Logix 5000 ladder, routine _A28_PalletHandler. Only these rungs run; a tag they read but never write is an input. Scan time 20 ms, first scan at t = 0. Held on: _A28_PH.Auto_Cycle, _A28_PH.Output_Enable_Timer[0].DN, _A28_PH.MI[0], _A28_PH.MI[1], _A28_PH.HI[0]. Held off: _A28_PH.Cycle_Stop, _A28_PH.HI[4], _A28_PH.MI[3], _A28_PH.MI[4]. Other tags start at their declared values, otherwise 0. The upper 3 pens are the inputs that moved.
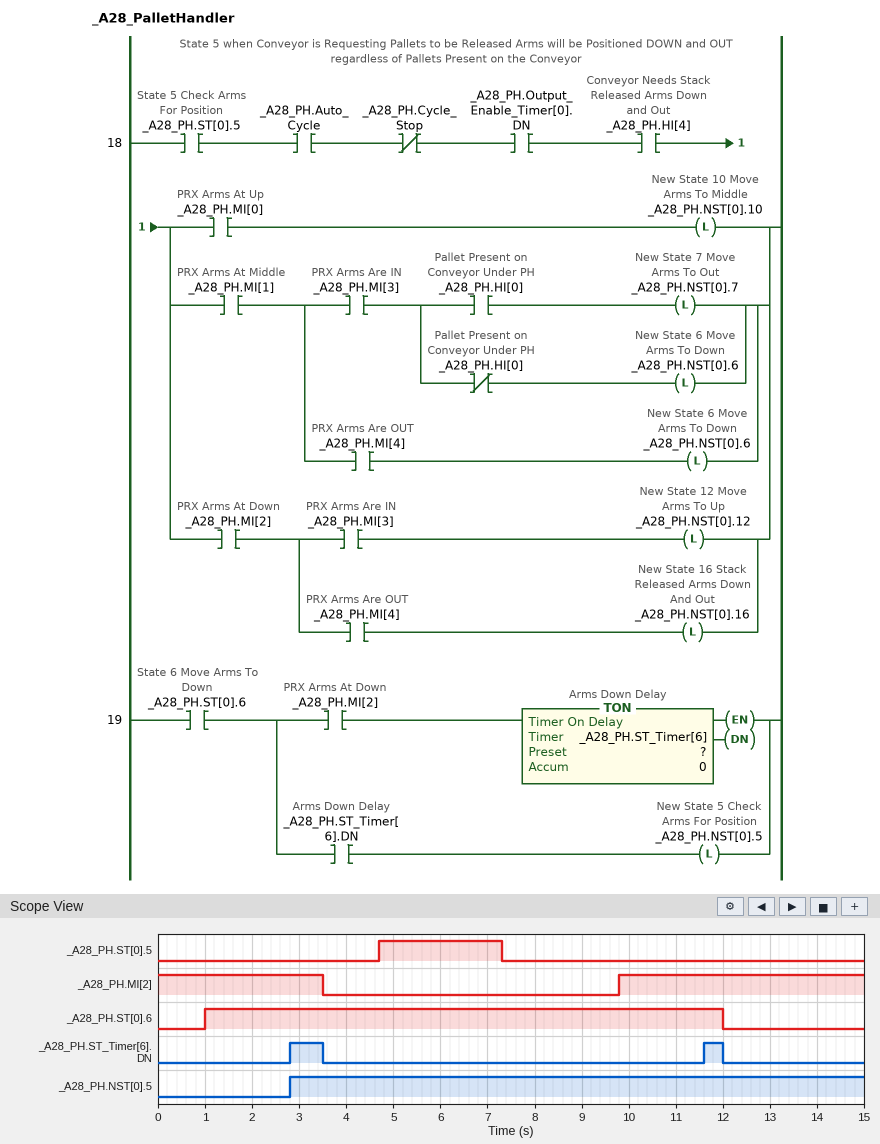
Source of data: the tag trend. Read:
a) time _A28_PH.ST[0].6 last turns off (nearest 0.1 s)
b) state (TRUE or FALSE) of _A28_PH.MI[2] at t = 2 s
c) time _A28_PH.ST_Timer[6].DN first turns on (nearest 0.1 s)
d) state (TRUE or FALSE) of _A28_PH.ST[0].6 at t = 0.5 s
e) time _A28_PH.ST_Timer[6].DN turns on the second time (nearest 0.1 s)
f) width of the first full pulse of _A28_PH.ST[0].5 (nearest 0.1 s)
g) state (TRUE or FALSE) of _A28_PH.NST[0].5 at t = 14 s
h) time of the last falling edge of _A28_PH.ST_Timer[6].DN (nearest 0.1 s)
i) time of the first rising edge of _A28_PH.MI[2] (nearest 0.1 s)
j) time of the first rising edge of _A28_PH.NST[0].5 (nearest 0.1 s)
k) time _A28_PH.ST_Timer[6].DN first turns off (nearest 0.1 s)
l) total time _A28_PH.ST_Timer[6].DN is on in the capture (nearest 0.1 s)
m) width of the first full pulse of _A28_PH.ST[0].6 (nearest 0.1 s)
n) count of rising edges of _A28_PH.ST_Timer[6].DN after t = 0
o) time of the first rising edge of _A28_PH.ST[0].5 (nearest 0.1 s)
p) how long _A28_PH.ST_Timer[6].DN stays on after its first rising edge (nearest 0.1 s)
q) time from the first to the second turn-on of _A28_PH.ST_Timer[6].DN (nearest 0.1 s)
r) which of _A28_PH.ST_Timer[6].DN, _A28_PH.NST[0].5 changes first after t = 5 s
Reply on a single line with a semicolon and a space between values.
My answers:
12.0 s; TRUE; 2.8 s; FALSE; 11.6 s; 2.6 s; TRUE; 12.0 s; 9.8 s; 2.8 s; 3.5 s; 1.1 s; 11.0 s; 2; 4.7 s; 0.7 s; 8.8 s; _A28_PH.ST_Timer[6].DN
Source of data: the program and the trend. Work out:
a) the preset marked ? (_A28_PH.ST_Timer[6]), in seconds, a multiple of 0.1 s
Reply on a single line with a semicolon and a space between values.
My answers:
1.8 s
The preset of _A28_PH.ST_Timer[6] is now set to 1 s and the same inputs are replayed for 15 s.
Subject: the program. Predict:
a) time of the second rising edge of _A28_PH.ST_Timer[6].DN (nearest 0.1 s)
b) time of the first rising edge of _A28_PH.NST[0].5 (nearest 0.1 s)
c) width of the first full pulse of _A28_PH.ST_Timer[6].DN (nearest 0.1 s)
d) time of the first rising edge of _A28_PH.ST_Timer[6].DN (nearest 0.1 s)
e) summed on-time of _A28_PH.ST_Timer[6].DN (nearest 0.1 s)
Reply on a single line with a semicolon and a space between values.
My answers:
10.8 s; 2.0 s; 1.5 s; 2.0 s; 2.7 s
